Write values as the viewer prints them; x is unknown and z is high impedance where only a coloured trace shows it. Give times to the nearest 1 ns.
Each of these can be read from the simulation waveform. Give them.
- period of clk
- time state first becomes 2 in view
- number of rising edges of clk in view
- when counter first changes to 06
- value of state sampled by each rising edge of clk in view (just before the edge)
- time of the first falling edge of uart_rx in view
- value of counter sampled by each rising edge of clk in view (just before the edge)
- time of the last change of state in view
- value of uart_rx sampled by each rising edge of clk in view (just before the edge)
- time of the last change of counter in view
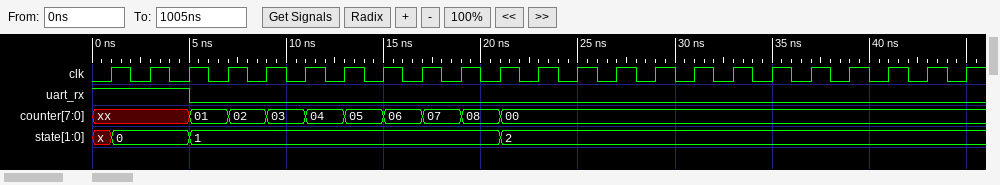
2 ns
21 ns
23
15 ns
x, 0, 0, 1, 1, 1, 1, 1, 1, 1, 1, 2, 2, 2, 2, 2, 2, 2, 2, 2, 2, 2, 2
5 ns
xx, xx, xx, 01, 02, 03, 04, 05, 06, 07, 08, 00, 00, 00, 00, 00, 00, 00, 00, 00, 00, 00, 00
21 ns
1 1 1 0 0 0 0 0 0 0 0 0 0 0 0 0 0 0 0 0 0 0 0
21 ns
